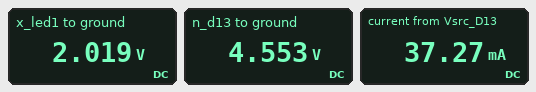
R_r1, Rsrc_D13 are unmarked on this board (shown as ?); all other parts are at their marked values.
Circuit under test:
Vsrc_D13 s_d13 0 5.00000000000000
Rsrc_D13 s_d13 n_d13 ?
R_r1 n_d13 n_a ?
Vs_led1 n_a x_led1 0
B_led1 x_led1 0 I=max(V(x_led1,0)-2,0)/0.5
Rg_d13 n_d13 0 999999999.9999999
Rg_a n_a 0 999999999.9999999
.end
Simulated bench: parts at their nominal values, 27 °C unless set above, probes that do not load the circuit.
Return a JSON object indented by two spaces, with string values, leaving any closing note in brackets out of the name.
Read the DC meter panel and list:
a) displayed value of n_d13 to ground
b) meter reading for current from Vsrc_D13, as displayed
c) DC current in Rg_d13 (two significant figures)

{
  "displayed value of n_d13 to ground": "4.553 V",
  "meter reading for current from Vsrc_D13, as displayed": "37.27 mA",
  "DC current in Rg_d13": "4.6 nA"
}
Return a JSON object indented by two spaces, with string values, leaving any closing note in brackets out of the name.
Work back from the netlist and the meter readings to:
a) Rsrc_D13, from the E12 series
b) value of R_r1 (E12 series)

{
  "Rsrc_D13, from the E12 series": "12 Ω",
  "value of R_r1": "68 Ω"
}
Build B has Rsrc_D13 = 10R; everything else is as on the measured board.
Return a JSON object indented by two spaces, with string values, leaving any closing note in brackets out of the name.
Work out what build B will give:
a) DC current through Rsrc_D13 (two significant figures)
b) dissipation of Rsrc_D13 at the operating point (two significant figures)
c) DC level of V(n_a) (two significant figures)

{
  "DC current through Rsrc_D13": "38 mA",
  "dissipation of Rsrc_D13 at the operating point": "15 mW",
  "DC level of V(n_a)": "2.0 V"
}
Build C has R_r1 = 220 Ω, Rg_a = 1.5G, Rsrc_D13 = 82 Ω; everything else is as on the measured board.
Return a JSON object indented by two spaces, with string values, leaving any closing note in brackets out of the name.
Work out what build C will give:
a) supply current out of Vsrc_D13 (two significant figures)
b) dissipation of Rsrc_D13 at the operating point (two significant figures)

{
  "supply current out of Vsrc_D13": "9.9 mA",
  "dissipation of Rsrc_D13 at the operating point": "8.1 mW"
}
